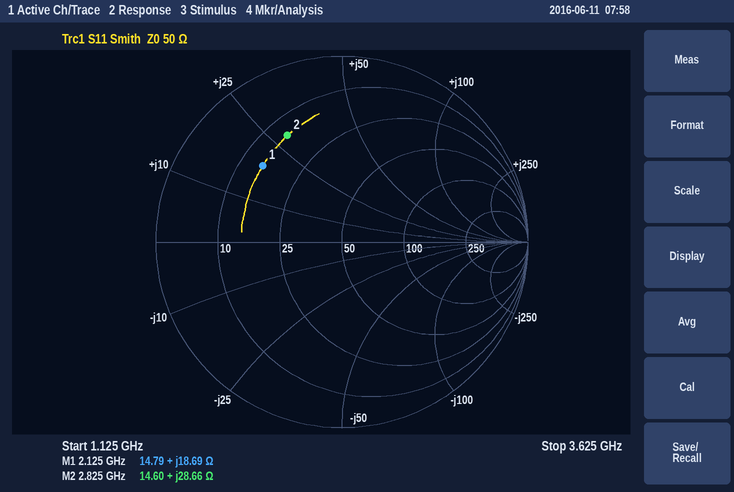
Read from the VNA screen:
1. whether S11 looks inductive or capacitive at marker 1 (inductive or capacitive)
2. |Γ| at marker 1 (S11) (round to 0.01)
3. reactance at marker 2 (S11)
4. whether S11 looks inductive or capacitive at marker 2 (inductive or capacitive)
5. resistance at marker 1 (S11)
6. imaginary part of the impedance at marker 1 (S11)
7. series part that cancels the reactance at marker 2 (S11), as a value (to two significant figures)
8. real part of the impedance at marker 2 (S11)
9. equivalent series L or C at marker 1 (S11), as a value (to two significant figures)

inductive
0.59
+28.66 Ω
inductive
14.79 Ω
+18.69 Ω
2.0 pF
14.60 Ω
1.4 nH
